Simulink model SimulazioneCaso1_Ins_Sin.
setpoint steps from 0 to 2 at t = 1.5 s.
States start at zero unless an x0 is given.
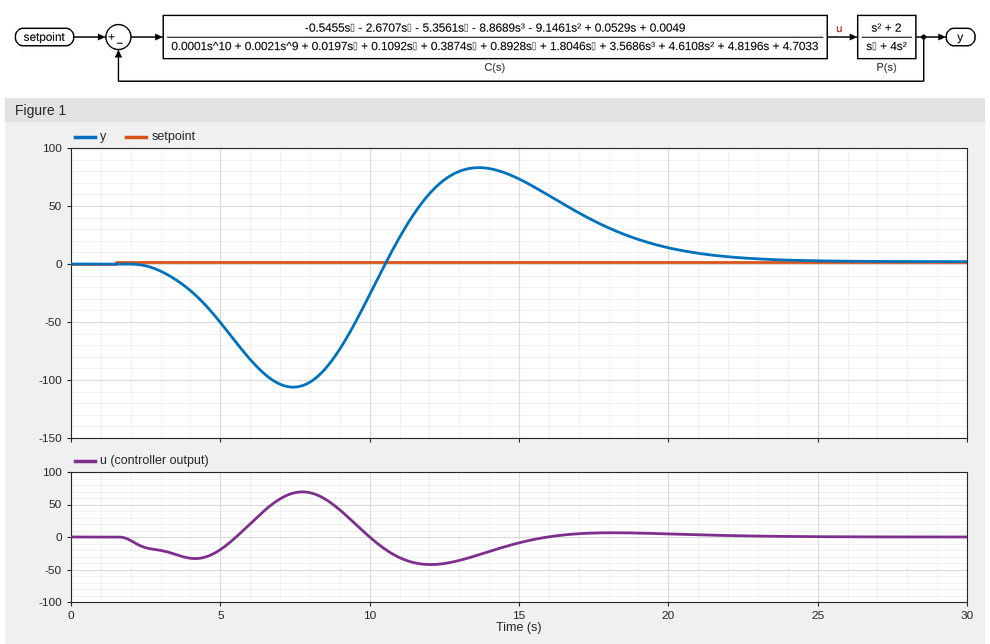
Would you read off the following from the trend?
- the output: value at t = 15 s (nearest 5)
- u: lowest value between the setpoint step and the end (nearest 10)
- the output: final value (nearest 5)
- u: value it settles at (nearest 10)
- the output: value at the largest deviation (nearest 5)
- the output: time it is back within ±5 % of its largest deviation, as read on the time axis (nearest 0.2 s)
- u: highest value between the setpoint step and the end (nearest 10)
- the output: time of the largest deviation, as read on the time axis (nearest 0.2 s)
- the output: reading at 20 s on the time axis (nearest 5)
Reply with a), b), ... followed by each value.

a) 75
b) -40
c) 0
d) 0
e) -105
f) 21.6 s
g) 70
h) 7.4 s
i) 15
